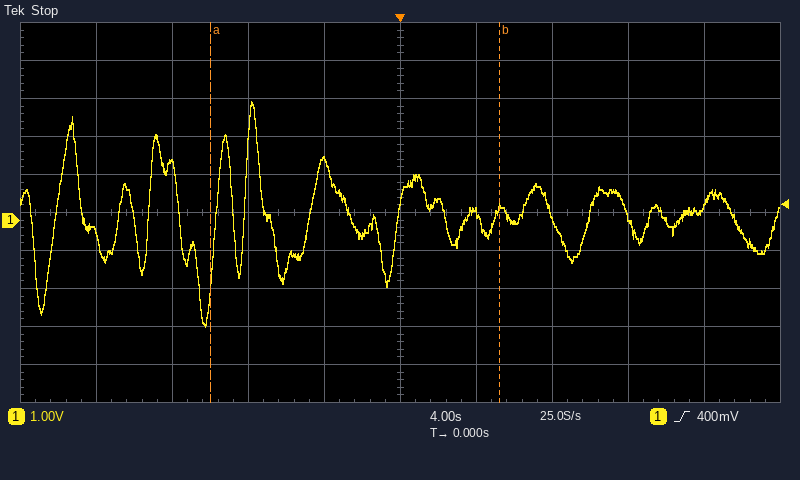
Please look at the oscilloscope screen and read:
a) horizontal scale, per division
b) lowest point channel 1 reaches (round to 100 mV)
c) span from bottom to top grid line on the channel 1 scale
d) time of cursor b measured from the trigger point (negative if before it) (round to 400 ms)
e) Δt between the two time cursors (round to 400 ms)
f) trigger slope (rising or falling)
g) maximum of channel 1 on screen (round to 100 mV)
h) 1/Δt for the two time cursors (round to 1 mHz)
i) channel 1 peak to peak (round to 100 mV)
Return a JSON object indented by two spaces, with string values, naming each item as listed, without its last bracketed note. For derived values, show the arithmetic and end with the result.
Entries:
{
  "horizontal scale, per division": "4 s",
  "lowest point channel 1 reaches": "-2.8 V",
  "span from bottom to top grid line on the channel 1 scale": "10 V",
  "time of cursor b measured from the trigger point (negative if before it)": "+5.2 s",
  "Δt between the two time cursors": "15.2 s",
  "trigger slope": "rising",
  "maximum of channel 1 on screen": "3.1 V",
  "1/Δt for the two time cursors": "1 / 15.2 s ≈ 66 mHz",
  "channel 1 peak to peak": "3.1 V − (-2.8 V) = 5.9 V"
}
